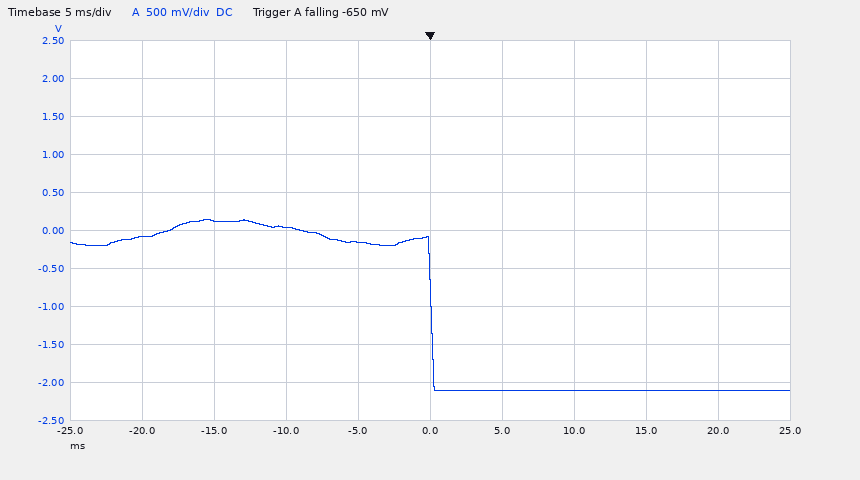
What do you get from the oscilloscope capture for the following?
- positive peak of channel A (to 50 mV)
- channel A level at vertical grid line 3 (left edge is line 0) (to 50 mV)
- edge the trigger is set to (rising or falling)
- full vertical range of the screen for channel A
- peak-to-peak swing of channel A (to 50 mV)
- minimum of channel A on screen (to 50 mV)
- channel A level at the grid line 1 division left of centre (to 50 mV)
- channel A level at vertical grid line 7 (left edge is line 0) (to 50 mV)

150 mV
50 mV
falling
5 V
2.25 V
-2.10 V
-150 mV
-2.10 V
